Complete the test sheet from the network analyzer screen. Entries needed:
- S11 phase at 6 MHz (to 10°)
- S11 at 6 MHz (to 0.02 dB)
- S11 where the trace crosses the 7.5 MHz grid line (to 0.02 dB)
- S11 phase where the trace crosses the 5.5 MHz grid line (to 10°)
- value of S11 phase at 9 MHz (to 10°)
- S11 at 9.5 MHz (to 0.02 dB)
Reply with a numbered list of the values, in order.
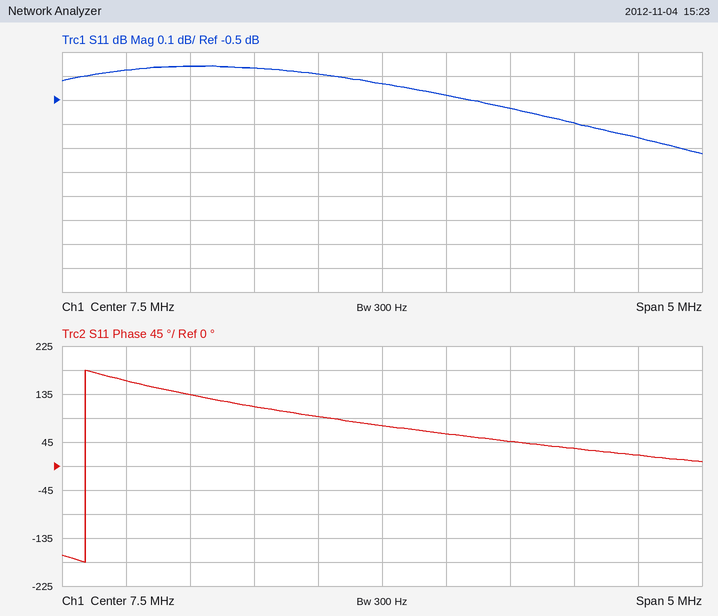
1. 130°
2. -0.36 dB
3. -0.44 dB
4. 160°
5. 30°
6. -0.66 dB
